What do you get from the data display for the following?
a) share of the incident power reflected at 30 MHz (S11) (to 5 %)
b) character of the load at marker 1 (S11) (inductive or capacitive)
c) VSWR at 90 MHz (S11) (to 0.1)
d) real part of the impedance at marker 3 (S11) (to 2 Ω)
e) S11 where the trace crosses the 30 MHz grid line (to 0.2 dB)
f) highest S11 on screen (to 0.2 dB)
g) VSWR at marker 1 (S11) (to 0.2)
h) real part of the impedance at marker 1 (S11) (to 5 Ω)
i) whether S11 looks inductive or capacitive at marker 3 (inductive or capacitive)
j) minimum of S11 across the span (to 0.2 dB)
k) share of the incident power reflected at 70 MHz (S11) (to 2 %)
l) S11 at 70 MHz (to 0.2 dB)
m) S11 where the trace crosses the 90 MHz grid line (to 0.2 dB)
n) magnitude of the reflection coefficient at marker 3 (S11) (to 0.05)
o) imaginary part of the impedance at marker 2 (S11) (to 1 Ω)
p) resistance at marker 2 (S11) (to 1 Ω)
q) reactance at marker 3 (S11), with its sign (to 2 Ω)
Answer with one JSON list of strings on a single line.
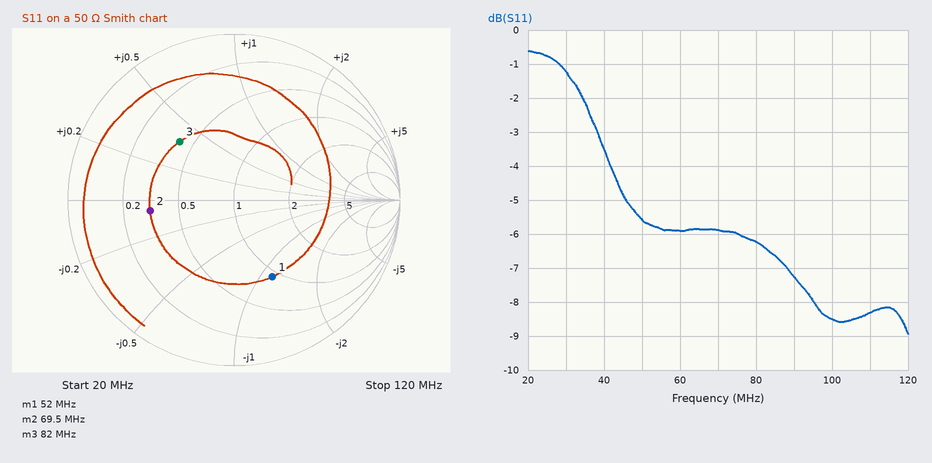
["75 %", "capacitive", "2.5", "20 Ω", "-1.2 dB", "-0.6 dB", "3.2", "45 Ω", "inductive", "-9.0 dB", "26 %", "-5.8 dB", "-7.2 dB", "0.50", "-3 Ω", "16 Ω", "+18 Ω"]
